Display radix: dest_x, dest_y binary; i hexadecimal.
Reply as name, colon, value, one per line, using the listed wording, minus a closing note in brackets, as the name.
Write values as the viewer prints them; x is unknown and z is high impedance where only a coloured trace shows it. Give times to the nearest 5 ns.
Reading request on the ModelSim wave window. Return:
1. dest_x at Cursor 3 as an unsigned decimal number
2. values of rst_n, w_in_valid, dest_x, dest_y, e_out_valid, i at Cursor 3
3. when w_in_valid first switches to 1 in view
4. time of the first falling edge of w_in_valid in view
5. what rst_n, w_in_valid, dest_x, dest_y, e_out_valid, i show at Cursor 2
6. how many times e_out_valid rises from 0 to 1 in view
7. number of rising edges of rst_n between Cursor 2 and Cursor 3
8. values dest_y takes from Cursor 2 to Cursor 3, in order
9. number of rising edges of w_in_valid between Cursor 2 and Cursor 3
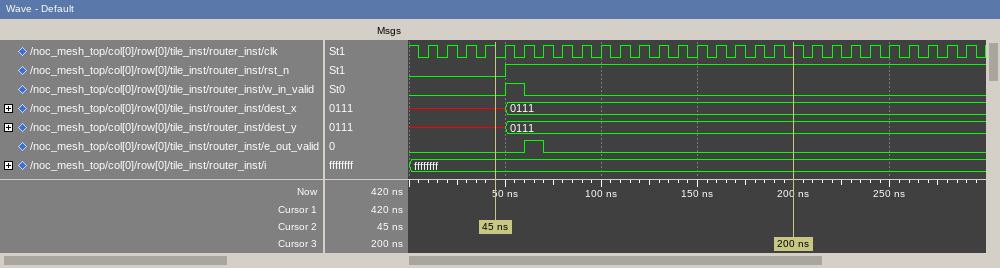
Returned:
dest_x at Cursor 3 as an unsigned decimal number: 7
values of rst_n, w_in_valid, dest_x, dest_y, e_out_valid, i at Cursor 3: rst_n=1, w_in_valid=0, dest_x=0111, dest_y=0111, e_out_valid=0, i=ffffffff
when w_in_valid first switches to 1 in view: 50 ns
time of the first falling edge of w_in_valid in view: 60 ns
what rst_n, w_in_valid, dest_x, dest_y, e_out_valid, i show at Cursor 2: rst_n=0, w_in_valid=0, dest_x=x, dest_y=x, e_out_valid=0, i=ffffffff
how many times e_out_valid rises from 0 to 1 in view: 1
number of rising edges of rst_n between Cursor 2 and Cursor 3: 1
values dest_y takes from Cursor 2 to Cursor 3, in order: x, 0111
number of rising edges of w_in_valid between Cursor 2 and Cursor 3: 1
